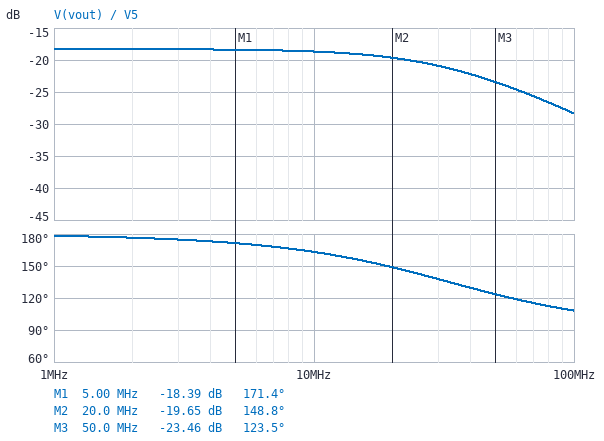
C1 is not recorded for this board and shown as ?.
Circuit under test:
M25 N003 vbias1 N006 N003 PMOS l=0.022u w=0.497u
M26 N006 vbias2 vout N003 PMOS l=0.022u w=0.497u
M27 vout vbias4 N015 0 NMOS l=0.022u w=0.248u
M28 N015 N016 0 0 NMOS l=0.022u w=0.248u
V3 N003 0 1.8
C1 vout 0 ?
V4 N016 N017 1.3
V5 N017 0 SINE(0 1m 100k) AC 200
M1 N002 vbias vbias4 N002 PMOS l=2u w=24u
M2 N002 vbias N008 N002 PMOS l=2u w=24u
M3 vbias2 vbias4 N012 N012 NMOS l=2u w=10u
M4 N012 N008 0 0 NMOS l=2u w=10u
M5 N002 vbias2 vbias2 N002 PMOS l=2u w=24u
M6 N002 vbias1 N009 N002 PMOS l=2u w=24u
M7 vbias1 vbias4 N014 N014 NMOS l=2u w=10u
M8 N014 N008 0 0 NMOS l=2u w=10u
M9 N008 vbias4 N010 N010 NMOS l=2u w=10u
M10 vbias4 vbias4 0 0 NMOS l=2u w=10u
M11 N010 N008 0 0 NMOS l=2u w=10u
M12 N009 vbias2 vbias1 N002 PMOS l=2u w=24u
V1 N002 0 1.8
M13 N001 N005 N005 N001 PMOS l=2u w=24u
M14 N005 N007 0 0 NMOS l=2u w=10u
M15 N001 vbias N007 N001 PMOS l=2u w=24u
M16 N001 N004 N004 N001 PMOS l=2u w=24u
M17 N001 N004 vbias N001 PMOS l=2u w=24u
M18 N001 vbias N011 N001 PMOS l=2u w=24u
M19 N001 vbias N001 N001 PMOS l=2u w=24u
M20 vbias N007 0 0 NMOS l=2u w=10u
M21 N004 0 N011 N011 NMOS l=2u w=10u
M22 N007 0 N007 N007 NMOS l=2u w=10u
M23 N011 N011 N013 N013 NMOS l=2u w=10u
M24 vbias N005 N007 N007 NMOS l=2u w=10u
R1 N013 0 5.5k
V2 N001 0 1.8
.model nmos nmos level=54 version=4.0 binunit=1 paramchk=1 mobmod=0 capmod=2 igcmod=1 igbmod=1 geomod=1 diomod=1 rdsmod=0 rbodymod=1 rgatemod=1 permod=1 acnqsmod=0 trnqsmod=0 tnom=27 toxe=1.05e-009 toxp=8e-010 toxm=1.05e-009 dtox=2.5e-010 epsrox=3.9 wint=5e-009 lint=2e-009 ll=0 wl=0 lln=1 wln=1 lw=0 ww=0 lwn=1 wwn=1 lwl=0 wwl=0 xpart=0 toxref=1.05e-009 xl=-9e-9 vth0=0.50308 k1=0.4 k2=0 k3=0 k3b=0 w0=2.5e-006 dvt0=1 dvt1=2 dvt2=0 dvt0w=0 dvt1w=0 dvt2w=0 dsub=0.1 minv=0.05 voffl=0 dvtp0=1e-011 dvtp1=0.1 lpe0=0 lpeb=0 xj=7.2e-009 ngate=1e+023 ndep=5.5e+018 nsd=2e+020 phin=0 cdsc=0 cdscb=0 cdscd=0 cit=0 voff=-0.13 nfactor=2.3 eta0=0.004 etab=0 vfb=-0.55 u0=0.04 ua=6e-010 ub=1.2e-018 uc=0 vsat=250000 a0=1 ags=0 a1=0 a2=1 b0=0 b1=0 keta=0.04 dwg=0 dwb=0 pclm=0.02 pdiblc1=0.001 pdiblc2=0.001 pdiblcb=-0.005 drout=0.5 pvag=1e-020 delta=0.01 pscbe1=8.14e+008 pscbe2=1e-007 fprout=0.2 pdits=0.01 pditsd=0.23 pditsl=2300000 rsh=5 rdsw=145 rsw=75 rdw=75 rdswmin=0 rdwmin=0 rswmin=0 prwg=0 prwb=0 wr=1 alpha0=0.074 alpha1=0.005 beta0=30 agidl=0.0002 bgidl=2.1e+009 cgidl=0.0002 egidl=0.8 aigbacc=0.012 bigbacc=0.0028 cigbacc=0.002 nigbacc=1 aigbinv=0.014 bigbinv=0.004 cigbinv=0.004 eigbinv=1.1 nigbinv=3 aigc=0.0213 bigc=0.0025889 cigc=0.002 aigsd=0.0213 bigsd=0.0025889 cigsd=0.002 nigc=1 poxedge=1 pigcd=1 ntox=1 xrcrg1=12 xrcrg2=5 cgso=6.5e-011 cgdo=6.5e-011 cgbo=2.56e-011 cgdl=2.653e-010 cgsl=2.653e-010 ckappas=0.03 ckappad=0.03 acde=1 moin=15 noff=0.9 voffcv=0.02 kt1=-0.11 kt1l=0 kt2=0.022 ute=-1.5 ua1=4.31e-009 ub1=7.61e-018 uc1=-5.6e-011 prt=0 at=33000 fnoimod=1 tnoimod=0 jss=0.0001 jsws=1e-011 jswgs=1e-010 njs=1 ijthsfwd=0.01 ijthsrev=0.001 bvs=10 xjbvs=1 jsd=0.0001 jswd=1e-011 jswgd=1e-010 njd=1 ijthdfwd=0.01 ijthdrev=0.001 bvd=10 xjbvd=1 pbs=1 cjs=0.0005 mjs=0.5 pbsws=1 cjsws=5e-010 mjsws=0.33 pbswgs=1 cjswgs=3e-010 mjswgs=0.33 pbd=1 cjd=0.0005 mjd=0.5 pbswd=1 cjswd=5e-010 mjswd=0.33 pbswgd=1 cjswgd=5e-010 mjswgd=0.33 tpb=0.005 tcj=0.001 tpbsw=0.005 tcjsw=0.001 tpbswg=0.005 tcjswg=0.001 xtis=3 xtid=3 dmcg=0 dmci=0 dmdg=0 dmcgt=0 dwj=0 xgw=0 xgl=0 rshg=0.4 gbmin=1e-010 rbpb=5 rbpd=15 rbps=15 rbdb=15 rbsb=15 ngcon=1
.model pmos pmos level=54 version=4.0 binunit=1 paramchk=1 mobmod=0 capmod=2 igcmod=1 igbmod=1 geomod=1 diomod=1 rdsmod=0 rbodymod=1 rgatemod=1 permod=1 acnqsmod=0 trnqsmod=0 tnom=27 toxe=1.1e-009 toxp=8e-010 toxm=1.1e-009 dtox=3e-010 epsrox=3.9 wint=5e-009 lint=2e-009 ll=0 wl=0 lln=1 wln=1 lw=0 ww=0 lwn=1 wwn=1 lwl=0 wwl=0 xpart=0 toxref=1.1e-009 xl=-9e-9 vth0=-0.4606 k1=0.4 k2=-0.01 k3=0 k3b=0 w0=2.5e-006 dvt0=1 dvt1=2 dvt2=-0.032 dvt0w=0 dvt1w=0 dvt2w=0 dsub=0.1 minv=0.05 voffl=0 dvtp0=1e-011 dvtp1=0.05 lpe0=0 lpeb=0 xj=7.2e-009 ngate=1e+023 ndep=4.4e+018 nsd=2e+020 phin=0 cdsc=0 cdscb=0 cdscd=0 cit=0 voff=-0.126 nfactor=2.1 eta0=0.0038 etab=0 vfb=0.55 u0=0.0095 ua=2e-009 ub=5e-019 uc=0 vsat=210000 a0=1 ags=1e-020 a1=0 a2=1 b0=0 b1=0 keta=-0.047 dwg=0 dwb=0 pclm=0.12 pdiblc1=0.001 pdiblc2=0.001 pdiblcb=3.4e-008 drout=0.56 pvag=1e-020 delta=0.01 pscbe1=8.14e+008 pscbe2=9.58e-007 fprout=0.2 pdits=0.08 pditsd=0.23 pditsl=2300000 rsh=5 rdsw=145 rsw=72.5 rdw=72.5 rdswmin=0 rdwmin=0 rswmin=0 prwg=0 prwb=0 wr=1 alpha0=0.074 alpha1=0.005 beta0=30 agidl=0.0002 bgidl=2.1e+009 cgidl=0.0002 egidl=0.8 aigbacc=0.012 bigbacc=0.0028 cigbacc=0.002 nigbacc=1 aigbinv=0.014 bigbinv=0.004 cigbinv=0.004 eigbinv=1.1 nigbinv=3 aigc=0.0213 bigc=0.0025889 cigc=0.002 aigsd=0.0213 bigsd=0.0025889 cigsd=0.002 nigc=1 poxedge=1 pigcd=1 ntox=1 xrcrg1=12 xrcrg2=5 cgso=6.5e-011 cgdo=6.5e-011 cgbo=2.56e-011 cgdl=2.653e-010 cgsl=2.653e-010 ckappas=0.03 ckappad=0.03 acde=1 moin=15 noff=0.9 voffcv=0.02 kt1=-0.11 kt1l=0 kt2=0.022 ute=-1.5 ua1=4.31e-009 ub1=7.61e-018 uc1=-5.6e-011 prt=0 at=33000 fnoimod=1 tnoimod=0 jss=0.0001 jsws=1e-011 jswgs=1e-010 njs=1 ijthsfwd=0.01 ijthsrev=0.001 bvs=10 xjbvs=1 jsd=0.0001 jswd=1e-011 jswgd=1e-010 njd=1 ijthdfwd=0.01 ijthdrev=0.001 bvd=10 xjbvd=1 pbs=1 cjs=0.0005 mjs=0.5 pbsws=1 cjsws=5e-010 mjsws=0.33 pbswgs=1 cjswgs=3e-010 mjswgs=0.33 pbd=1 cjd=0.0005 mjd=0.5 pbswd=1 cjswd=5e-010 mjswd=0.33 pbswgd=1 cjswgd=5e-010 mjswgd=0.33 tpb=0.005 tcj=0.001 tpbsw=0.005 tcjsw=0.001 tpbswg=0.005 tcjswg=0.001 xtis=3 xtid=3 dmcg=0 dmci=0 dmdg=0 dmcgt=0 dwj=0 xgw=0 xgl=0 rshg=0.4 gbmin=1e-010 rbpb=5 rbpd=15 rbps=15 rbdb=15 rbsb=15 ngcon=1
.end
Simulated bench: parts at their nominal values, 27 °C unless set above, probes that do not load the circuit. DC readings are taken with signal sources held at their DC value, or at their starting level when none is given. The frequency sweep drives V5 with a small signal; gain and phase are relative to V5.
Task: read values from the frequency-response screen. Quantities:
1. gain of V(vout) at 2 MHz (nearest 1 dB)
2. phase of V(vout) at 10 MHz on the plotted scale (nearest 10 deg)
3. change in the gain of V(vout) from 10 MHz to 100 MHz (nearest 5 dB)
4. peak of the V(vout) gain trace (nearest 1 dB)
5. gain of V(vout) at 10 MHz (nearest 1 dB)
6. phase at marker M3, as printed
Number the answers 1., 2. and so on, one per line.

1. -18 dB
2. 160 deg
3. -10 dB
4. -18 dB
5. -19 dB
6. 123.5 deg
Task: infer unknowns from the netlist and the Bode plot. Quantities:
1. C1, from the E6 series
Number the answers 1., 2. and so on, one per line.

1. 1.5 pF
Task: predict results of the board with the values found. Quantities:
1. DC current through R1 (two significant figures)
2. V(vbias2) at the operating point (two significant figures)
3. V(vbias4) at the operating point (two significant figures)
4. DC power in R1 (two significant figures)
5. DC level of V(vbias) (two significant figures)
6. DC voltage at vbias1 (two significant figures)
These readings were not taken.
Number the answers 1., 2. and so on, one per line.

1. 43 µA
2. 810 mV
3. 990 mV
4. 10 µW
5. 610 mV
6. 580 mV
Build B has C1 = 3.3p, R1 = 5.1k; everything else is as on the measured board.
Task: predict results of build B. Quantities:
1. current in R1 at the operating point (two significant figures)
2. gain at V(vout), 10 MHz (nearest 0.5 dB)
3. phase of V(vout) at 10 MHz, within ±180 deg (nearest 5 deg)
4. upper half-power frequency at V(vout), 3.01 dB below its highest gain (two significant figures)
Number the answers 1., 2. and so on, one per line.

1. 45 µA
2. -20.0 dB
3. 145 deg
4. 15 MHz
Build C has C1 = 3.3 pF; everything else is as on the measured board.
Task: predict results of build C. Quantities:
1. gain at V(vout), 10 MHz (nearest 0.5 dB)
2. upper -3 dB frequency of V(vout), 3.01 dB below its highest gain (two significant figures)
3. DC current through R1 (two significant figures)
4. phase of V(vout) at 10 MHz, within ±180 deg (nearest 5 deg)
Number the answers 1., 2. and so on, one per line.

1. -20.0 dB
2. 15 MHz
3. 43 µA
4. 145 deg
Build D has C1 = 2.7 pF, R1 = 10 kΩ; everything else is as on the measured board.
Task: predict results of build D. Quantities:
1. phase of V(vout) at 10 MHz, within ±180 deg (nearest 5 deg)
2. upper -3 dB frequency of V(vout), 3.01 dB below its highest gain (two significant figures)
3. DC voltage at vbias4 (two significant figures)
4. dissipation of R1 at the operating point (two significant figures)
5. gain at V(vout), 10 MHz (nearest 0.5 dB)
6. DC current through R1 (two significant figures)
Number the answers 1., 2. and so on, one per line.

1. 150 deg
2. 18 MHz
3. 990 mV
4. 8.2 µW
5. -19.5 dB
6. 29 µA
